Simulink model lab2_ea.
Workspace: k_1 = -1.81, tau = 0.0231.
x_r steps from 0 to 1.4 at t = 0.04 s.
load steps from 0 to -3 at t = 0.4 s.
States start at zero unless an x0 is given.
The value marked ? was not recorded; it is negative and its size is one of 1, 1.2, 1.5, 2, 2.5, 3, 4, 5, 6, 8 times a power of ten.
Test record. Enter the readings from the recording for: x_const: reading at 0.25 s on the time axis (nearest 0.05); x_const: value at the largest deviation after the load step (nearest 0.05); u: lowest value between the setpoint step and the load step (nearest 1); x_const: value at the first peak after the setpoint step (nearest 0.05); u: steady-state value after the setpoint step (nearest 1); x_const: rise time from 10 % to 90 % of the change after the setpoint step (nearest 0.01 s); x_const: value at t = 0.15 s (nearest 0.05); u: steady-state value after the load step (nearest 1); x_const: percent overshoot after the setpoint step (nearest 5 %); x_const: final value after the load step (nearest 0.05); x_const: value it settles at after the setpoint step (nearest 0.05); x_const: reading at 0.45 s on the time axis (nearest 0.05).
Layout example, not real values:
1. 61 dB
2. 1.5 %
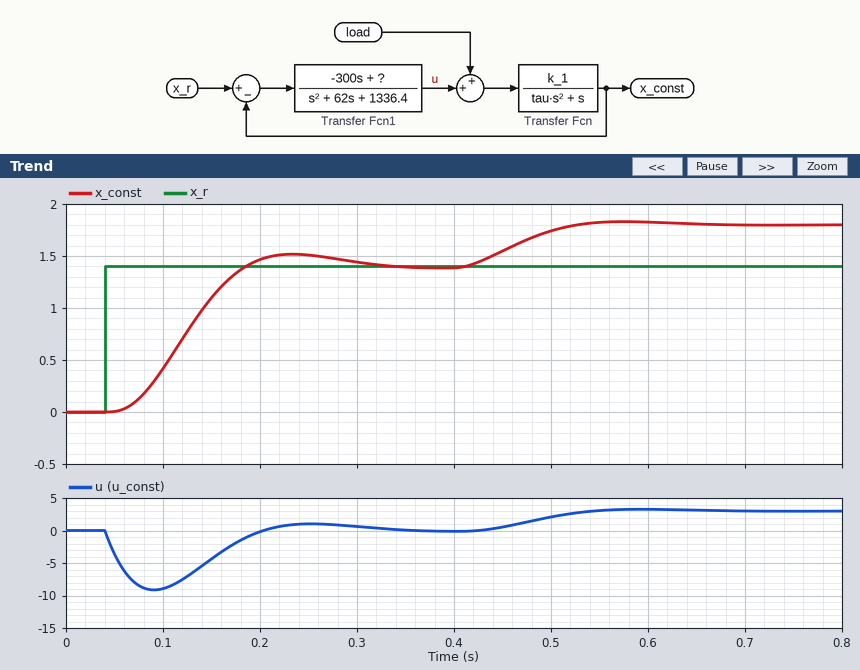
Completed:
1. 1.50
2. 1.85
3. -9
4. 1.50
5. 0
6. 0.09 s
7. 1.10
8. 3
9. 10 %
10. 1.80
11. 1.40
12. 1.55
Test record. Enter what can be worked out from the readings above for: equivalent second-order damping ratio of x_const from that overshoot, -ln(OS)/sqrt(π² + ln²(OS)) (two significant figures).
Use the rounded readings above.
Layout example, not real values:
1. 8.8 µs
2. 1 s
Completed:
1. 0.59
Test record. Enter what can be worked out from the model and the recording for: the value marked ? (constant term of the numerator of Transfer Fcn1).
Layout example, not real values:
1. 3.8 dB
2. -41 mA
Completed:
1. -10000
